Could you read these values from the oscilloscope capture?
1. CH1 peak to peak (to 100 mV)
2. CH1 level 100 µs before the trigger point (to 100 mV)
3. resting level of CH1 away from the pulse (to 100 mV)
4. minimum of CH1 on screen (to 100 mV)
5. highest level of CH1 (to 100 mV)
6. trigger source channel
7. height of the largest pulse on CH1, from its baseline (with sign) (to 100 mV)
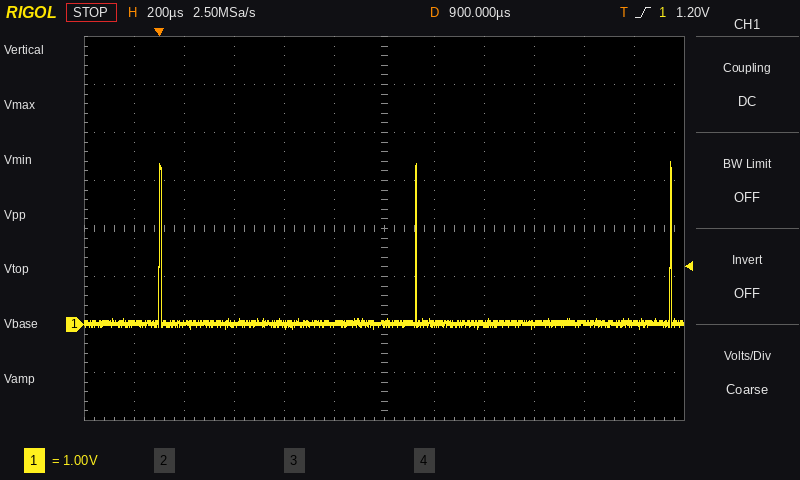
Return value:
3.5 V
0.0 V
0.0 V
-100 mV
3.4 V
CH1
+3.4 V
